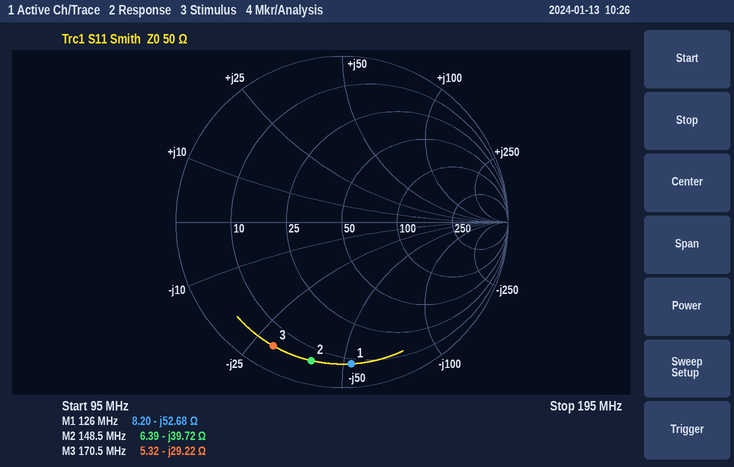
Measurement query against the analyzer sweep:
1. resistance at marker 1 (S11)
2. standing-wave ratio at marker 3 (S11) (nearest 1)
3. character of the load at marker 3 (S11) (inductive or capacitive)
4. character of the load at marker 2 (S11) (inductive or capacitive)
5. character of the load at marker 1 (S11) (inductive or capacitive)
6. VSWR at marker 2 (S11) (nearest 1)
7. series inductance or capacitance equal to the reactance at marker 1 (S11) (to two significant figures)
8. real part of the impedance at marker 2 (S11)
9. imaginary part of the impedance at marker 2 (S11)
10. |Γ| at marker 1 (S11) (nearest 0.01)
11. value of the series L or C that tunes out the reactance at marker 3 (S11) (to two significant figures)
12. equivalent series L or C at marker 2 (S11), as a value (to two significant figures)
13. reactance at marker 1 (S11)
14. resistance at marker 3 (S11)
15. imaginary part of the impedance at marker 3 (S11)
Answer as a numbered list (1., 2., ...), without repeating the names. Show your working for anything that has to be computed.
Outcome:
1. 8.20 Ω
2. 13
3. capacitive
4. capacitive
5. capacitive
6. 13
7. C = 1/(2π × 126 MHz × 52.68 Ω) ≈ 24 pF
8. 6.39 Ω
9. -39.72 Ω
10. 0.86
11. L = 29.22 Ω/(2π × 170.5 MHz) ≈ 27 nH
12. C = 1/(2π × 148.5 MHz × 39.72 Ω) ≈ 27 pF
13. -52.68 Ω
14. 5.32 Ω
15. -29.22 Ω
